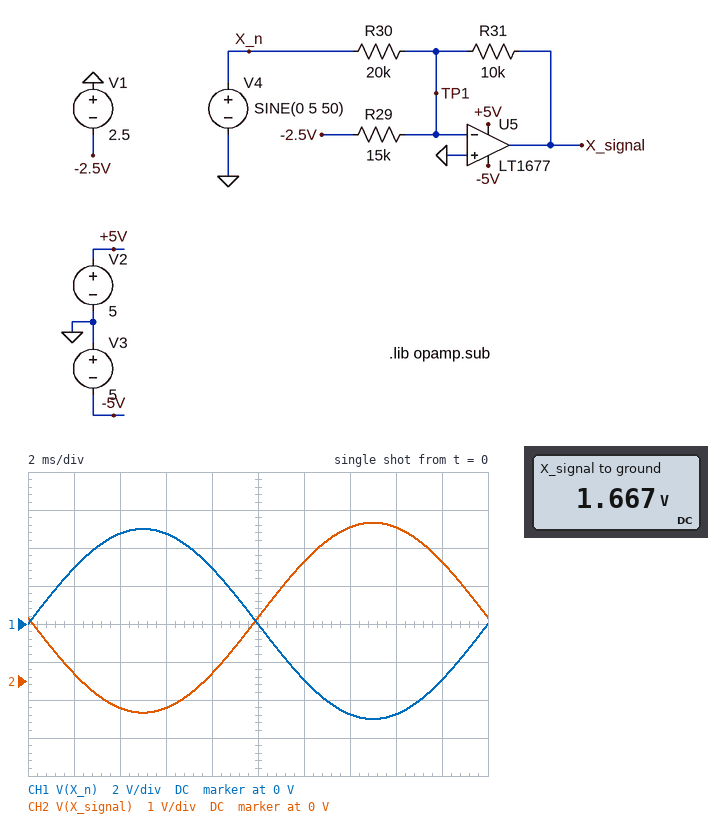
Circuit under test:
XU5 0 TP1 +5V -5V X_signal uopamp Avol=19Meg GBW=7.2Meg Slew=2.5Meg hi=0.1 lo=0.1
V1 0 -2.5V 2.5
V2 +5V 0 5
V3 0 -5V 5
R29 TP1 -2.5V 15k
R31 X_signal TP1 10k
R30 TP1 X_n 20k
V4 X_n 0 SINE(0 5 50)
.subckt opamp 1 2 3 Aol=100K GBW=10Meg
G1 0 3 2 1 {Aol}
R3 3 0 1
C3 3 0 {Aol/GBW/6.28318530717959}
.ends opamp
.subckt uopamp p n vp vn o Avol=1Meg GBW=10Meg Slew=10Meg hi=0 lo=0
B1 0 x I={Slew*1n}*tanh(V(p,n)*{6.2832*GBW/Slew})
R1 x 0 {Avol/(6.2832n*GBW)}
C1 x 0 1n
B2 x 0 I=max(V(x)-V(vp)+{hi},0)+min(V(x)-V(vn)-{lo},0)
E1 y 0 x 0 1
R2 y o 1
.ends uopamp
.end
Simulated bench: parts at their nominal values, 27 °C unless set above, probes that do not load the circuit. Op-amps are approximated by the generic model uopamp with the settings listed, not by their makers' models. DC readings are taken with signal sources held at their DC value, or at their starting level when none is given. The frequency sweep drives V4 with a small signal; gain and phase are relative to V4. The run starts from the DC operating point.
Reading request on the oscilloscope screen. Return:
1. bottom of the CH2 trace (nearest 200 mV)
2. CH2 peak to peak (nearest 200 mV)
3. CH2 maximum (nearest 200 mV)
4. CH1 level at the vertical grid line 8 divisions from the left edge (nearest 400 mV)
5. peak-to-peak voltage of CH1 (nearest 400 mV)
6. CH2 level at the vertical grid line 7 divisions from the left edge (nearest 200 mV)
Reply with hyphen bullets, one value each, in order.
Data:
- -800 mV
- 5.0 V
- 4.2 V
- -4.8 V
- 10.0 V
- 4.0 V
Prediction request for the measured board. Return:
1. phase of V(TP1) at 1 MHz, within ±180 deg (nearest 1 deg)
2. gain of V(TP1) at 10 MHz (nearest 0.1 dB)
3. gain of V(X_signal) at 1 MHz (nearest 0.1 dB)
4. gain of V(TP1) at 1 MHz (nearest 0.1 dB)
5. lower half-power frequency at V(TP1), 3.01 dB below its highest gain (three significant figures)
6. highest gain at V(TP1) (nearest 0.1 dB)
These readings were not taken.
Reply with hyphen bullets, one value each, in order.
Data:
- 73 deg
- -13.2 dB
- -6.4 dB
- -23.5 dB
- 3.32 MHz
- -12.7 dB
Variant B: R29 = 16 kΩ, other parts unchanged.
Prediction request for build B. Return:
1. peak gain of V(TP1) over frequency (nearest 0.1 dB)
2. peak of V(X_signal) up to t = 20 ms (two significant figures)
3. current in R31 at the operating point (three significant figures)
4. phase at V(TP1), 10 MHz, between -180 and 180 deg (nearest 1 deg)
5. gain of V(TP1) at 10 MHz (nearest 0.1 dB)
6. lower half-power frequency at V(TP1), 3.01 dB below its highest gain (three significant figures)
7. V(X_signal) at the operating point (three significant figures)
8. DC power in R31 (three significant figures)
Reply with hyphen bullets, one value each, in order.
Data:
- -12.6 dB
- 4.1 V
- 156 µA
- 19 deg
- -13.0 dB
- 3.39 MHz
- 1.56 V
- 244 µW
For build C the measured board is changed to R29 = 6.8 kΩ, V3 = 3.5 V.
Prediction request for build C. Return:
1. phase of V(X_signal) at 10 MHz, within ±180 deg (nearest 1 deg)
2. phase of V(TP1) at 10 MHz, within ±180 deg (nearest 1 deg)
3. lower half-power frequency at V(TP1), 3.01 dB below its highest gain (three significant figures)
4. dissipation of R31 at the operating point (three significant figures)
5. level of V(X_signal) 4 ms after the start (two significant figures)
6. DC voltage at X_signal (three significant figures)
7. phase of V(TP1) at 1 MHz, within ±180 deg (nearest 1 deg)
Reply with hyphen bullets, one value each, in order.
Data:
- 104 deg
- 14 deg
- 2.42 MHz
- 1.35 mW
- 1.3 V
- 3.68 V
- 68 deg
